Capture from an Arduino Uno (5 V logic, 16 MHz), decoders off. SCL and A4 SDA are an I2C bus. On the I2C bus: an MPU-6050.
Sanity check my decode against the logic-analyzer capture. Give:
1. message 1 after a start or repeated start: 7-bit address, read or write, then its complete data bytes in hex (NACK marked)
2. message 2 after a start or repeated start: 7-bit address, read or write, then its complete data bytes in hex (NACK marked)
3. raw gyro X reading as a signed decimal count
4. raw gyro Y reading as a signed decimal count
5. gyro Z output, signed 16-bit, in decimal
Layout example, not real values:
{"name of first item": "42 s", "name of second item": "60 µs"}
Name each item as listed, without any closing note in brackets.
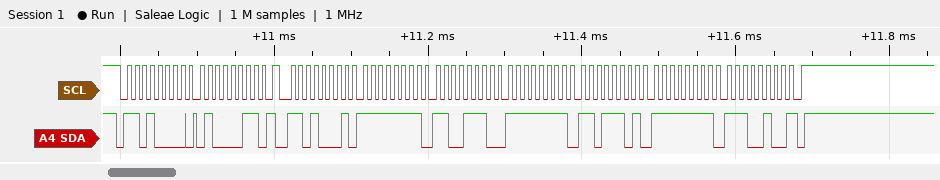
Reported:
{"message 1 after a start or repeated start: 7-bit address, read or write, then its complete data bytes in hex": "0x68 write: 43", "message 2 after a start or repeated start: 7-bit address, read or write, then its complete data bytes in hex": "0x68 read: FF CE FF DD FF E4 NACK", "raw gyro X reading as a signed decimal count": "-50", "raw gyro Y reading as a signed decimal count": "-35", "gyro Z output, signed 16-bit, in decimal": "-28"}
